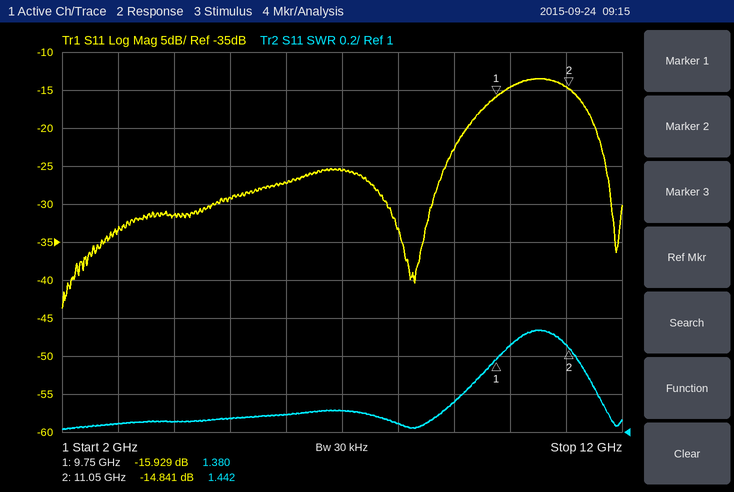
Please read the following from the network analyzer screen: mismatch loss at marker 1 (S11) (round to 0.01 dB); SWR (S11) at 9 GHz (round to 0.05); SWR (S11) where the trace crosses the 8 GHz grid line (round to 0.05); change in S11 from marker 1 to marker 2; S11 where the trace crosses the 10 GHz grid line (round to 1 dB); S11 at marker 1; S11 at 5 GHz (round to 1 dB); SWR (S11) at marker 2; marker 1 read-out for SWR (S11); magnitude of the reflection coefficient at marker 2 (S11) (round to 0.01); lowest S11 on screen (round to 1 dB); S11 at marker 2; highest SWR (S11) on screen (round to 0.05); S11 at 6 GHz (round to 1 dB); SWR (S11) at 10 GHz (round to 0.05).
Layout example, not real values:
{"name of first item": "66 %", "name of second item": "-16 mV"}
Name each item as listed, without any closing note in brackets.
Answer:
{"mismatch loss at marker 1 (S11)": "0.11 dB", "SWR (S11) at 9 GHz": "1.15", "SWR (S11) where the trace crosses the 8 GHz grid line": "1.05", "change in S11 from marker 1 to marker 2": "1.088 dB", "S11 where the trace crosses the 10 GHz grid line": "-15 dB", "S11 at marker 1": "-15.929 dB", "S11 at 5 GHz": "-29 dB", "SWR (S11) at marker 2": "1.442", "marker 1 read-out for SWR": "1.380", "magnitude of the reflection coefficient at marker 2 (S11)": "0.18", "lowest S11 on screen": "-44 dB", "S11 at marker 2": "-14.841 dB", "highest SWR (S11) on screen": "1.55", "S11 at 6 GHz": "-27 dB", "SWR (S11) at 10 GHz": "1.45"}
